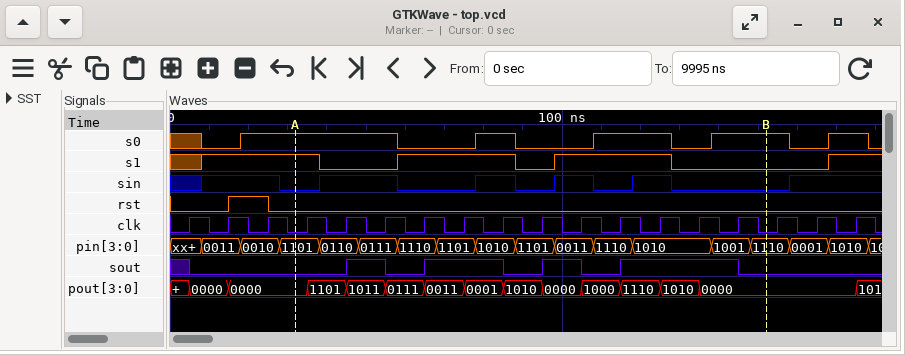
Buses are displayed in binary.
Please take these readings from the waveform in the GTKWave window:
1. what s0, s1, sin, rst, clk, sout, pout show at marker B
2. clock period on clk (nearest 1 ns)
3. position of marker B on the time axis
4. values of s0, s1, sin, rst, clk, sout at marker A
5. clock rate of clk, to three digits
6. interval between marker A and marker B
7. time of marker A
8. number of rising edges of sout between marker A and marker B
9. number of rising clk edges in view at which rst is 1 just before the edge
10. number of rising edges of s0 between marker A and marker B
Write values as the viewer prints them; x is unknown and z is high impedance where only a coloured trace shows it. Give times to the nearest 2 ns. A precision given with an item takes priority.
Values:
s0=1, s1=0, sin=0, rst=0, clk=0, sout=0, pout=0000
10 ns
152 ns
s0=1, s1=1, sin=0, rst=0, clk=0, sout=0
100 MHz
120 ns
32 ns
4
1
3
